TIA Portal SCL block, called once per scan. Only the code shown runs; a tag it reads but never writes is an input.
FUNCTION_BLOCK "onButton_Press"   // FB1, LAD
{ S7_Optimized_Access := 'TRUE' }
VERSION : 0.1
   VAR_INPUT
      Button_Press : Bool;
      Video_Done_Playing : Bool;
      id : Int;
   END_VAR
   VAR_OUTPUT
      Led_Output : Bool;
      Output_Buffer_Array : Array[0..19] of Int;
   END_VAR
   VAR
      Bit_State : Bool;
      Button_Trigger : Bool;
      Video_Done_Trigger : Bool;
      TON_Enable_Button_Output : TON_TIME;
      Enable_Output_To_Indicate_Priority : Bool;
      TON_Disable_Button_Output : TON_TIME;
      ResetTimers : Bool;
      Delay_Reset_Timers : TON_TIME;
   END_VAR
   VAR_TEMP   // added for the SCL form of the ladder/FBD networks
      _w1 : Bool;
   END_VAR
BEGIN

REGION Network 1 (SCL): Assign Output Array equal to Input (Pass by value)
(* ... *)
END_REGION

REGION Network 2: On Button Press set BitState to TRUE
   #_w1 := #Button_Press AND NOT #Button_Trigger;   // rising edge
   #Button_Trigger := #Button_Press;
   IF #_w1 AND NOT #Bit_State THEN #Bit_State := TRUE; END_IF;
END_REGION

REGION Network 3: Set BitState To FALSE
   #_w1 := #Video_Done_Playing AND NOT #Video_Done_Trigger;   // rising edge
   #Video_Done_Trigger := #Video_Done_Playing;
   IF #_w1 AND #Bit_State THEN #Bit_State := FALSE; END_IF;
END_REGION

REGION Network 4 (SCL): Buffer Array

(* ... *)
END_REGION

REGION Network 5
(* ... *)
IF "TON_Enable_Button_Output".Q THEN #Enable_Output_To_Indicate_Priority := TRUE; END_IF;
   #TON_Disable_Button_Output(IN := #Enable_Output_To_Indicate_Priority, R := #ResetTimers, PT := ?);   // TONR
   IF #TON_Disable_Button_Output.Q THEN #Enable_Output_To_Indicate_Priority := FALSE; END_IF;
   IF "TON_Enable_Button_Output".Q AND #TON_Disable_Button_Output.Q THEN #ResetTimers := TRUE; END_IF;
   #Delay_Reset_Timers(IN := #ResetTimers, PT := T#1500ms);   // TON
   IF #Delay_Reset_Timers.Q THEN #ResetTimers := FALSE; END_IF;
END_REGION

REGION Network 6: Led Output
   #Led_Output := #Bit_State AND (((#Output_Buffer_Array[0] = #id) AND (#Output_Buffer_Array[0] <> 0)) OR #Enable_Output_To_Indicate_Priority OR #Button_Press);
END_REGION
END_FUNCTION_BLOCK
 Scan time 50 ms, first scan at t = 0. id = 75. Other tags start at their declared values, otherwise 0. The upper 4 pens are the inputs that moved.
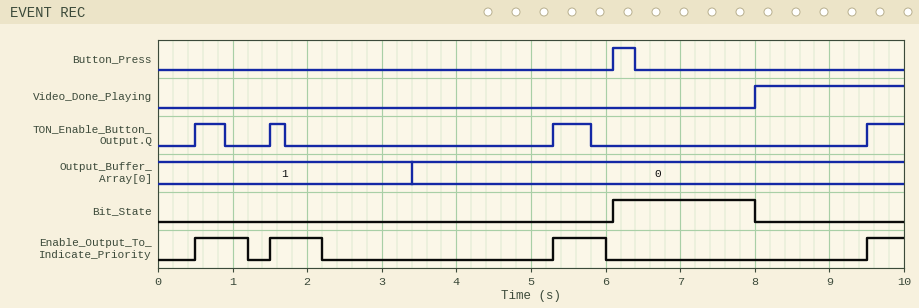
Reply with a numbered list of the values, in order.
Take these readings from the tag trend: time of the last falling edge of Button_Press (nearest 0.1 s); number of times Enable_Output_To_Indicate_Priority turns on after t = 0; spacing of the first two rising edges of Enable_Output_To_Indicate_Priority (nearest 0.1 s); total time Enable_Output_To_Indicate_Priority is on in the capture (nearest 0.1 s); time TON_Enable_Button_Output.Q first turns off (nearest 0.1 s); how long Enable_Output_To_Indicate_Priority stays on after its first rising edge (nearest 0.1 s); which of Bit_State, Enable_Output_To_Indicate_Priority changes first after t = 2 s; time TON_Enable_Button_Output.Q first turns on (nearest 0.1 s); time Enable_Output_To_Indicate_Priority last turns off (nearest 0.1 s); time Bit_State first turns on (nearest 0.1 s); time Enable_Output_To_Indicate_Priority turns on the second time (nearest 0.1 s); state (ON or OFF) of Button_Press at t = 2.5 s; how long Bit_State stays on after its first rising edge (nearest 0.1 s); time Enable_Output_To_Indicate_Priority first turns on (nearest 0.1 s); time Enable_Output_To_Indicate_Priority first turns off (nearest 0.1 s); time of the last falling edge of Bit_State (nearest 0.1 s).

1. 6.4 s
2. 4
3. 1.0 s
4. 2.6 s
5. 0.9 s
6. 0.7 s
7. Enable_Output_To_Indicate_Priority
8. 0.5 s
9. 6.0 s
10. 6.1 s
11. 1.5 s
12. OFF
13. 1.9 s
14. 0.5 s
15. 1.2 s
16. 8.0 s
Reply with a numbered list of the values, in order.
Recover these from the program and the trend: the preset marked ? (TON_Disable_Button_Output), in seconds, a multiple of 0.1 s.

1. 0.7 s
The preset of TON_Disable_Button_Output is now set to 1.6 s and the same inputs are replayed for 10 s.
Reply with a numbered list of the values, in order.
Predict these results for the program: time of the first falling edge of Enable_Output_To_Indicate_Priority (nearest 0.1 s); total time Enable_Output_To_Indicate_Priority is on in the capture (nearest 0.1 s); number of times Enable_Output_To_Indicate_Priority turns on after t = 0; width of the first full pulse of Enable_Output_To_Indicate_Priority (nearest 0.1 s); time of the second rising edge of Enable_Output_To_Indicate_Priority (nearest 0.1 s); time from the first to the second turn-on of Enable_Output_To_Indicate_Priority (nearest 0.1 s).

1. 2.1 s
2. 3.7 s
3. 3
4. 1.6 s
5. 5.3 s
6. 4.8 s
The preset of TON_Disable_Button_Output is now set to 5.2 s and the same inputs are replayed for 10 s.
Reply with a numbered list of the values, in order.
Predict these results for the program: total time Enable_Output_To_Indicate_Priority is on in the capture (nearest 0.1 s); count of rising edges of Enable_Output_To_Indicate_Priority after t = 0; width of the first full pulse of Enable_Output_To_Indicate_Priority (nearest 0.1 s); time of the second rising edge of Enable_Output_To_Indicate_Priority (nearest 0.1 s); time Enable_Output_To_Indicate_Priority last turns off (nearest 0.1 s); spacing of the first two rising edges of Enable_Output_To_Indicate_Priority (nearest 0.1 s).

1. 5.7 s
2. 2
3. 5.2 s
4. 9.5 s
5. 5.7 s
6. 9.0 s
